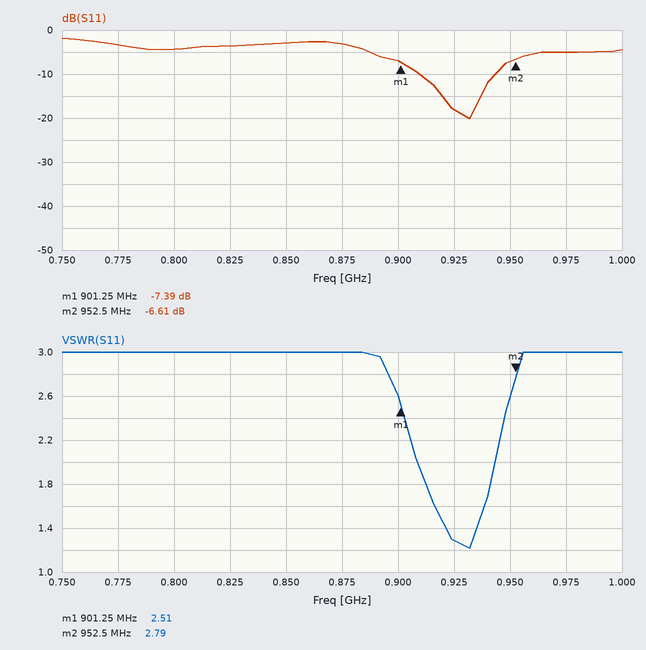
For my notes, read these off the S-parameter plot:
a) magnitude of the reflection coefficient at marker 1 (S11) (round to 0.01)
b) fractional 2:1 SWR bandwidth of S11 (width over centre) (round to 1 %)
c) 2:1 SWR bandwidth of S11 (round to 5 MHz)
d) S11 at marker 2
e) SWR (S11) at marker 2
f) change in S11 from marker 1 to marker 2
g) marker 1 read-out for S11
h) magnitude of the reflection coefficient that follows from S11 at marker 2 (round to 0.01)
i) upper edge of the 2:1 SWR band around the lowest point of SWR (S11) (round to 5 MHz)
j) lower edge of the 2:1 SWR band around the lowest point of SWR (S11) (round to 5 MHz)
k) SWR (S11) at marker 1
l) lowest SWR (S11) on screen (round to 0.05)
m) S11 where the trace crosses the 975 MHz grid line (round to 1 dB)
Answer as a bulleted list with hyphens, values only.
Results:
- 0.43
- 4 %
- 35 MHz
- -6.61 dB
- 2.79
- 0.78 dB
- -7.39 dB
- 0.47
- 945 MHz
- 910 MHz
- 2.51
- 1.20
- -5 dB
